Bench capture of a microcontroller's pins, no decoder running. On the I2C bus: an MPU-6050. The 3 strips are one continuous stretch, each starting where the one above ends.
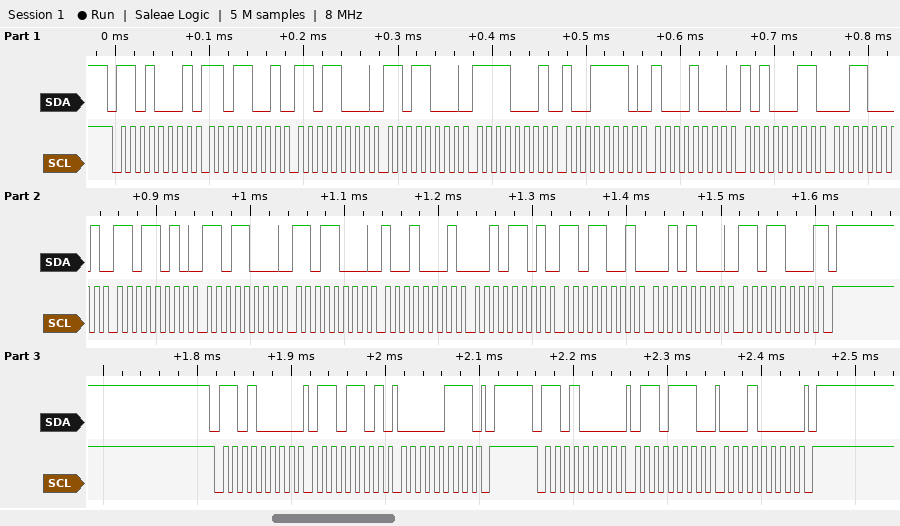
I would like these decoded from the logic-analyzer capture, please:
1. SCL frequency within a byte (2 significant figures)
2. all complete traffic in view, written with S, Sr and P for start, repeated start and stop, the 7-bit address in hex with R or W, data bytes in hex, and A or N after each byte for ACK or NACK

100 kHz
S 68R A D9 A D8 A D8 A F1 A 9E A 88 A A3 A 31 A DA A D8 A D8 A 91 A 2D A D9 A 28 A D8 N P S 68W A 6D A 07 A P S 68W A 6E A 10 A P
